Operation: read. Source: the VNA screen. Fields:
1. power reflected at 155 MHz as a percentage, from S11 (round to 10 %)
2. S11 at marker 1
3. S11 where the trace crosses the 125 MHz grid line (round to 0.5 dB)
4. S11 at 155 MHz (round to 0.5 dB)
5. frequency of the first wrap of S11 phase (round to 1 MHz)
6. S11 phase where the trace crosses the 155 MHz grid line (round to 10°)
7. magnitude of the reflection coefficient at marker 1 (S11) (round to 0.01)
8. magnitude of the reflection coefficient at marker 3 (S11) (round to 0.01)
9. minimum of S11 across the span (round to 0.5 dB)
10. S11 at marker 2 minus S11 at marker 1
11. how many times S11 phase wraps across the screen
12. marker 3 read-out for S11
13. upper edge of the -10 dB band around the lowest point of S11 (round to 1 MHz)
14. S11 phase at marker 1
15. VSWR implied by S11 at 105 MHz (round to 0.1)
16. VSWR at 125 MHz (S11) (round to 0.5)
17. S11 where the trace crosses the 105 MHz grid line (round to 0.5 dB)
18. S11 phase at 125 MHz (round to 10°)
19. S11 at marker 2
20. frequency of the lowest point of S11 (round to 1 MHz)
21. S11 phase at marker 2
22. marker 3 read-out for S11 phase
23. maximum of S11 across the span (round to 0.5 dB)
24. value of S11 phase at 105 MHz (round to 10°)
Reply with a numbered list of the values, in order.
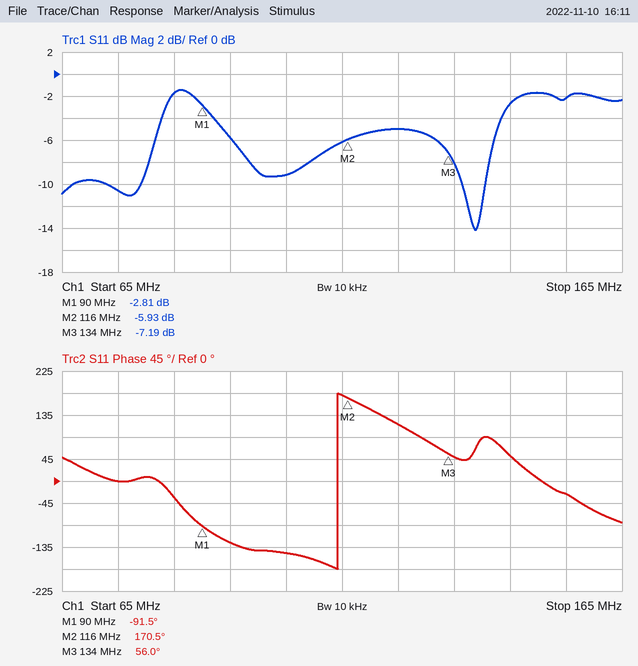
1. 60 %
2. -2.81 dB
3. -5.0 dB
4. -2.0 dB
5. 114 MHz
6. -30°
7. 0.72
8. 0.44
9. -14.0 dB
10. -3.12 dB
11. 1
12. -7.19 dB
13. 141 MHz
14. -91.5°
15. 2.1
16. 3.5
17. -9.0 dB
18. 120°
19. -5.93 dB
20. 139 MHz
21. 170.5°
22. 56.0°
23. -1.5 dB
24. -150°
